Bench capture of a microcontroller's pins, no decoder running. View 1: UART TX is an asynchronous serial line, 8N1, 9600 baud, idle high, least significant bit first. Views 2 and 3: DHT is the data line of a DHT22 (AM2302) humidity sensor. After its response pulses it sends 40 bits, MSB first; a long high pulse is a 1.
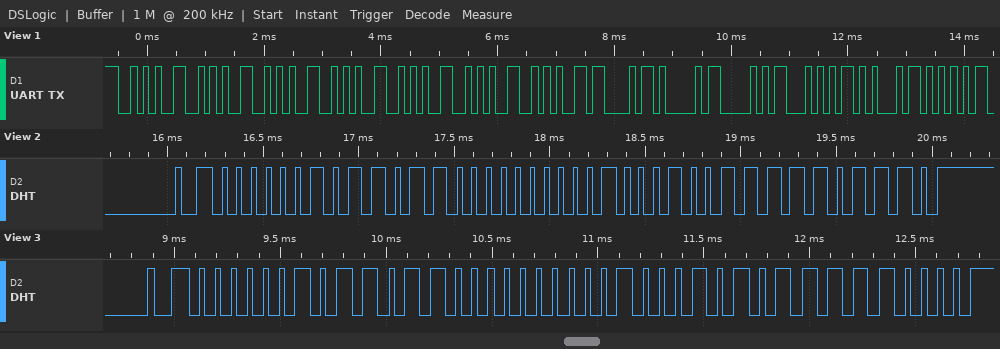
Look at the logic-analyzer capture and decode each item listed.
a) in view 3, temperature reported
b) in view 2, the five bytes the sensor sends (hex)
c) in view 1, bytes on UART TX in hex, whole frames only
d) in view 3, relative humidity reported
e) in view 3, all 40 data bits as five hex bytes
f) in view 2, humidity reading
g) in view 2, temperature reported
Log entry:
27.7 °C
02 D8 01 13 EE
2A 2A 2A 2A 2A 2A 2A 43 41 50 54 45 55
72.8 %
02 D8 01 15 F0
72.8 %
27.5 °C
